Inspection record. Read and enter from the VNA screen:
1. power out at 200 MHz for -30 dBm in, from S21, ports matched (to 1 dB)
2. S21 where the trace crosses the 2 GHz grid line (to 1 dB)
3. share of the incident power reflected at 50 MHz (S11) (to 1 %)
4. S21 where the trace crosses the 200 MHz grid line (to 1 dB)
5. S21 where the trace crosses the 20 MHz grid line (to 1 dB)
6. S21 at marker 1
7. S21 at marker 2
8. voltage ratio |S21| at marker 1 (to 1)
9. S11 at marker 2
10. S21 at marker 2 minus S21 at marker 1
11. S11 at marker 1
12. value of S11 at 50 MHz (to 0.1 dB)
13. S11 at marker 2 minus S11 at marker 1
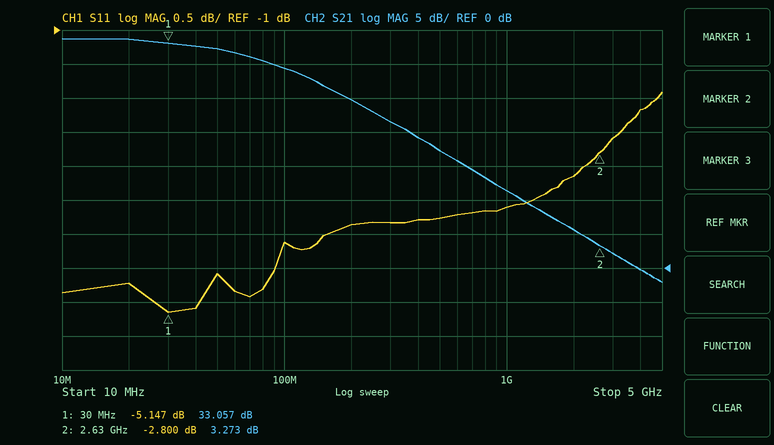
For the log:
-5 dBm
6 dB
35 %
25 dB
34 dB
33.057 dB
3.273 dB
45
-2.800 dB
-29.784 dB
-5.147 dB
-4.6 dB
2.347 dB
